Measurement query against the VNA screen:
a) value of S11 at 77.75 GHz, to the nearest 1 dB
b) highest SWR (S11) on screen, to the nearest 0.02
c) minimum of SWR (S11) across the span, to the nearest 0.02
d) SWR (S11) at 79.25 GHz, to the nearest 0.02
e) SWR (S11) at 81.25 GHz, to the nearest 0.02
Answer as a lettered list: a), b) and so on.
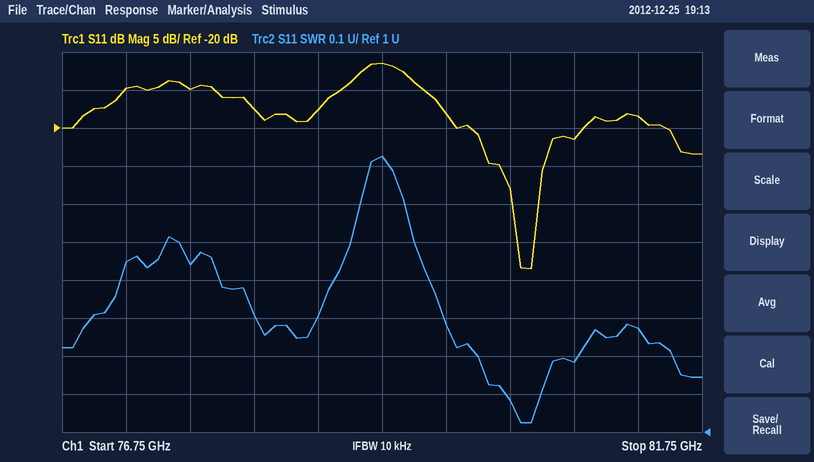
a) -15 dB
b) 1.72
c) 1.02
d) 1.72
e) 1.28
